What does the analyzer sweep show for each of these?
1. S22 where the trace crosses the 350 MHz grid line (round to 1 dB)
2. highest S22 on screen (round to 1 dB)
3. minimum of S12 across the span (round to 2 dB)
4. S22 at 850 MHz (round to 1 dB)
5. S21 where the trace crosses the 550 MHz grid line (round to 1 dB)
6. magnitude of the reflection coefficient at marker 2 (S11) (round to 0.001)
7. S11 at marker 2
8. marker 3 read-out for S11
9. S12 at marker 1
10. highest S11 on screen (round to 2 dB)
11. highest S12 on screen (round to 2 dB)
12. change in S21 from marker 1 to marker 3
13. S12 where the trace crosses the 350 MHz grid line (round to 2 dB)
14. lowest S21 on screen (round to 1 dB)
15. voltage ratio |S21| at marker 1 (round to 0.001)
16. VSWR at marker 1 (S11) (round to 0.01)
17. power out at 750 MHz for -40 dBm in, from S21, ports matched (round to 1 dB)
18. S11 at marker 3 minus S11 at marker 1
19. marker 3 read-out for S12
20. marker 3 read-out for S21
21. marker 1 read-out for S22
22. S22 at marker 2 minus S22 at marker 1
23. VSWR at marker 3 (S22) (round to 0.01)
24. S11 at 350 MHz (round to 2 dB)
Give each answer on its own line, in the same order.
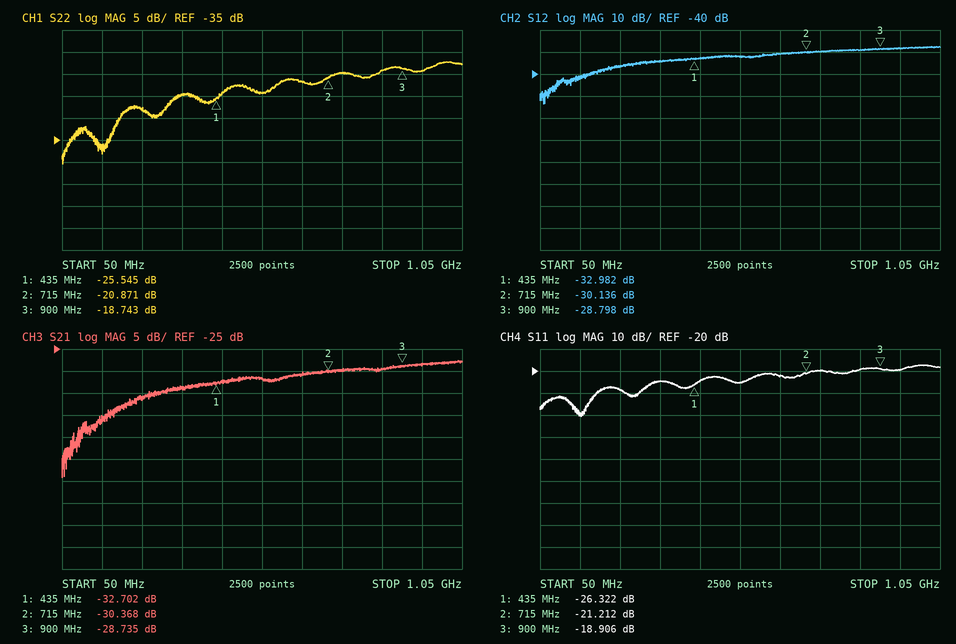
-25 dB
-17 dB
-54 dB
-19 dB
-32 dB
0.087
-21.212 dB
-18.906 dB
-32.982 dB
-18 dB
-28 dB
3.967 dB
-34 dB
-54 dB
0.023
1.10
-70 dBm
7.416 dB
-28.798 dB
-28.735 dB
-25.545 dB
4.674 dB
1.26
-24 dB
